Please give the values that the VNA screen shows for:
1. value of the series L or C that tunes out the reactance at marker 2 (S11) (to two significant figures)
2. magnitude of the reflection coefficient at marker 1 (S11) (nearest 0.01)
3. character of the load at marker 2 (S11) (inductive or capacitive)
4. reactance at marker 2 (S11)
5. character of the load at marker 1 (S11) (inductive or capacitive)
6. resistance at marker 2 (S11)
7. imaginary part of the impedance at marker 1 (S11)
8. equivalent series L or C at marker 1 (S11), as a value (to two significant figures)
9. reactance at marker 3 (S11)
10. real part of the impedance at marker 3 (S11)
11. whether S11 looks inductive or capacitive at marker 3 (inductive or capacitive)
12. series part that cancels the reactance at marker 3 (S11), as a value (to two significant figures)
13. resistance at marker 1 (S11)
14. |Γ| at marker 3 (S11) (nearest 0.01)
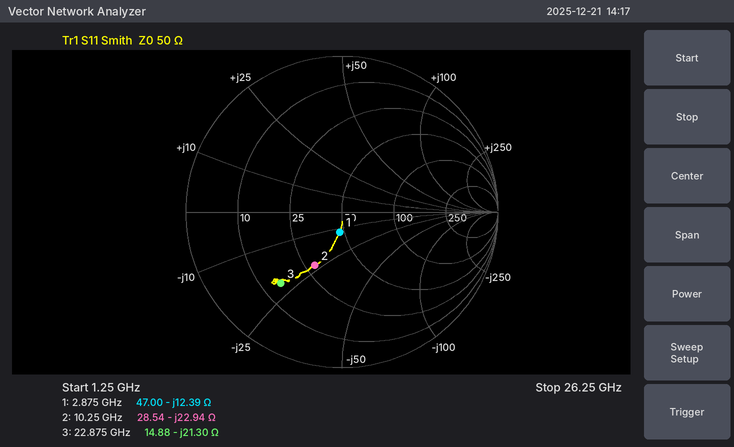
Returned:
360 pH
0.13
capacitive
-22.94 Ω
capacitive
28.54 Ω
-12.39 Ω
4.5 pF
-21.30 Ω
14.88 Ω
capacitive
150 pH
47.00 Ω
0.60
